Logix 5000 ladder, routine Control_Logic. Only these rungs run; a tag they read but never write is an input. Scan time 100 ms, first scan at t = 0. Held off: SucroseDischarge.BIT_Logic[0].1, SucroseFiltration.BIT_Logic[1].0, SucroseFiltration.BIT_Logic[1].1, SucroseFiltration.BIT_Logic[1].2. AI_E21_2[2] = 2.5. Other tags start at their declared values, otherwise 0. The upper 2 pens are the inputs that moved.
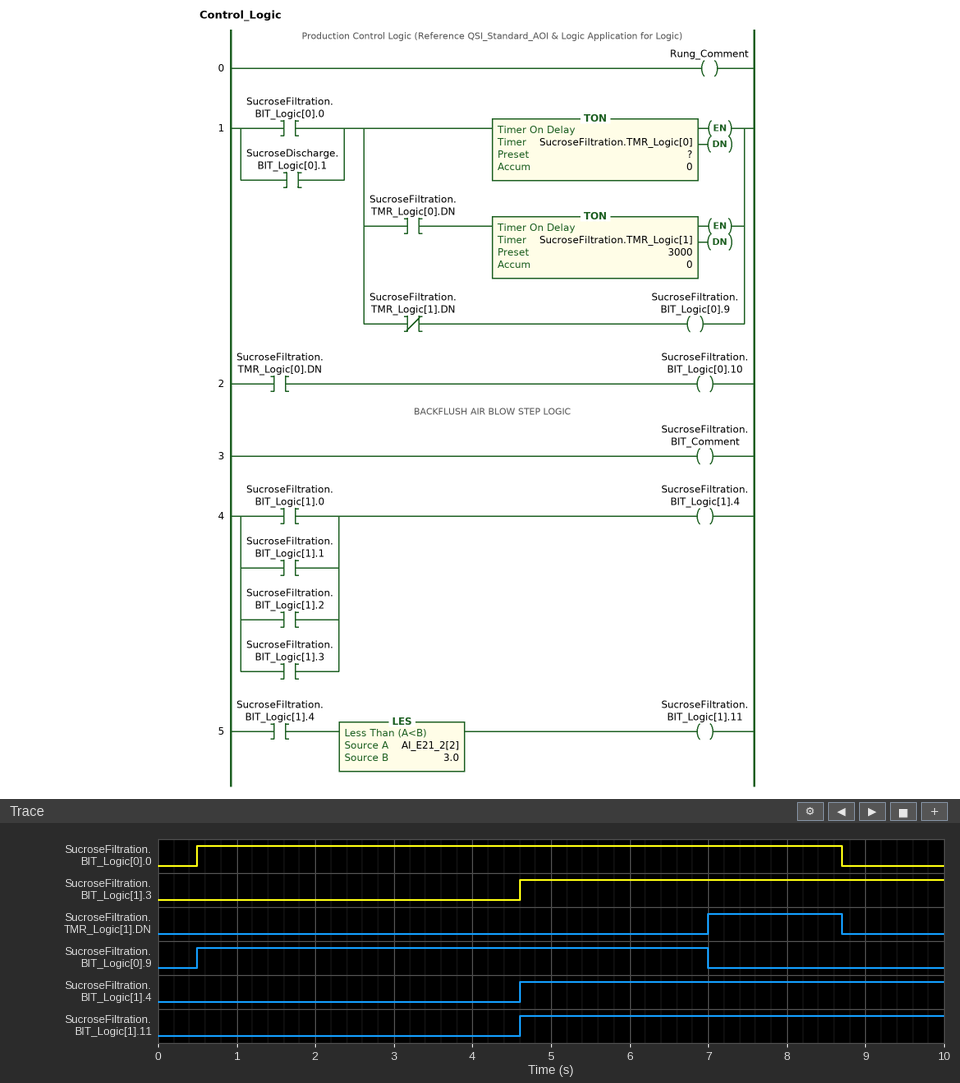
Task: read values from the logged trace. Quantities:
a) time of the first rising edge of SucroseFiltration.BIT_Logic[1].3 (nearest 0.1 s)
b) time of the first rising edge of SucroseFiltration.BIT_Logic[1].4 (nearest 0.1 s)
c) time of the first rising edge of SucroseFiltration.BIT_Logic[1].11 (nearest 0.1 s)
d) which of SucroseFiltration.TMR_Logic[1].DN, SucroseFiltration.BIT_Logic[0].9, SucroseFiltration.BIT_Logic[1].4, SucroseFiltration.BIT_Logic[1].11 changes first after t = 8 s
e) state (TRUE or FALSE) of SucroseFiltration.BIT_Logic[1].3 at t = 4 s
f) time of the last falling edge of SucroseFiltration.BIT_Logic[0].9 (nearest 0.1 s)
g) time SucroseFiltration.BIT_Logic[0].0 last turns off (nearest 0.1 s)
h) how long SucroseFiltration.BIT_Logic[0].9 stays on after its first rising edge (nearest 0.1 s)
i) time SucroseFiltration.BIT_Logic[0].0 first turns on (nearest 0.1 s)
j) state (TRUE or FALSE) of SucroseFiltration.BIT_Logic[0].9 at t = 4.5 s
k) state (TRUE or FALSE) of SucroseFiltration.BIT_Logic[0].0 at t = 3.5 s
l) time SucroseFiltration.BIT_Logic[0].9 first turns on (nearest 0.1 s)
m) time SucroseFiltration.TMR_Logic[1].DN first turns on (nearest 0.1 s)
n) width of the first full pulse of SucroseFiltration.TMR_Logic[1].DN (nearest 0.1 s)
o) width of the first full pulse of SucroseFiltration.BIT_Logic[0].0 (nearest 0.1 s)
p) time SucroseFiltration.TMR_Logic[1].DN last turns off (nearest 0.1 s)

4.6 s
4.6 s
4.6 s
SucroseFiltration.TMR_Logic[1].DN
FALSE
7.0 s
8.7 s
6.5 s
0.5 s
TRUE
TRUE
0.5 s
7.0 s
1.7 s
8.2 s
8.7 s
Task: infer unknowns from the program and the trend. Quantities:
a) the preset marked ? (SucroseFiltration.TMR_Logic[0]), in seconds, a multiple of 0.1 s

3.5 s
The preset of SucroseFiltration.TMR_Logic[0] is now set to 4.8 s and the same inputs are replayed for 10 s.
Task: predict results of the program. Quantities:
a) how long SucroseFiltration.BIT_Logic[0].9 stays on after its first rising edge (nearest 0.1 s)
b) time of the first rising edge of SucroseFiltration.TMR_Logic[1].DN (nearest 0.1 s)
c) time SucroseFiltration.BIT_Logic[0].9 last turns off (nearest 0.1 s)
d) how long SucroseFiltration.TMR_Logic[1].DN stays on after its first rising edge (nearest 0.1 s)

7.8 s
8.3 s
8.3 s
0.4 s
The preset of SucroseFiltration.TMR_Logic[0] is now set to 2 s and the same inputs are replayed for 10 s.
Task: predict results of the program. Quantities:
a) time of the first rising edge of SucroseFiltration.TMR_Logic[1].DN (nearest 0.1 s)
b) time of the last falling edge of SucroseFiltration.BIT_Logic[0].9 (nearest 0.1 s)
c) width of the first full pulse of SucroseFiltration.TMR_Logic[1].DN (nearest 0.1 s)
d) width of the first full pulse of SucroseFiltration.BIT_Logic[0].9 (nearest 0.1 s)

5.5 s
5.5 s
3.2 s
5.0 s
